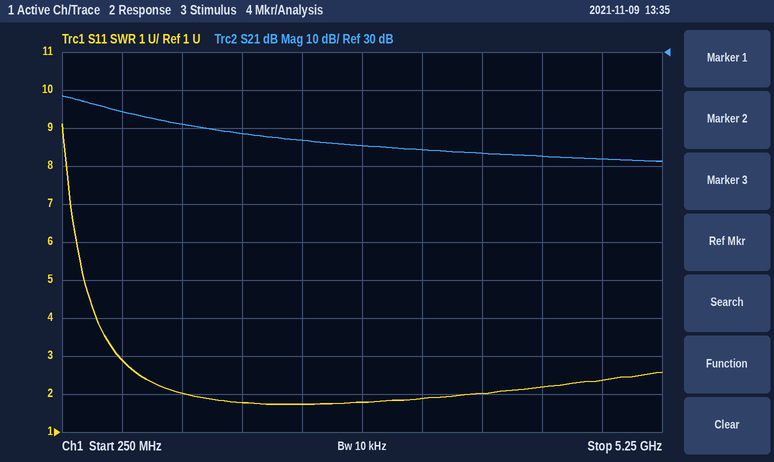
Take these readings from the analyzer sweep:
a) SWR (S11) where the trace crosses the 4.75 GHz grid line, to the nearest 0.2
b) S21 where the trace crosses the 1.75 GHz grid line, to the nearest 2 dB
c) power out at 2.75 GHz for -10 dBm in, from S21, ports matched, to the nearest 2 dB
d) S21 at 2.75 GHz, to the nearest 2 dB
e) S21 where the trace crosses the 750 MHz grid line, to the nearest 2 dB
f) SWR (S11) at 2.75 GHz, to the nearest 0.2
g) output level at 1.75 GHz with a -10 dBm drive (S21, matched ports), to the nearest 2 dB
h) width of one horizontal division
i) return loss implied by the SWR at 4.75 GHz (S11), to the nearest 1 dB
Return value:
2.4
8 dB
-4 dBm
6 dB
14 dB
1.8
-2 dBm
500 MHz
8 dB
